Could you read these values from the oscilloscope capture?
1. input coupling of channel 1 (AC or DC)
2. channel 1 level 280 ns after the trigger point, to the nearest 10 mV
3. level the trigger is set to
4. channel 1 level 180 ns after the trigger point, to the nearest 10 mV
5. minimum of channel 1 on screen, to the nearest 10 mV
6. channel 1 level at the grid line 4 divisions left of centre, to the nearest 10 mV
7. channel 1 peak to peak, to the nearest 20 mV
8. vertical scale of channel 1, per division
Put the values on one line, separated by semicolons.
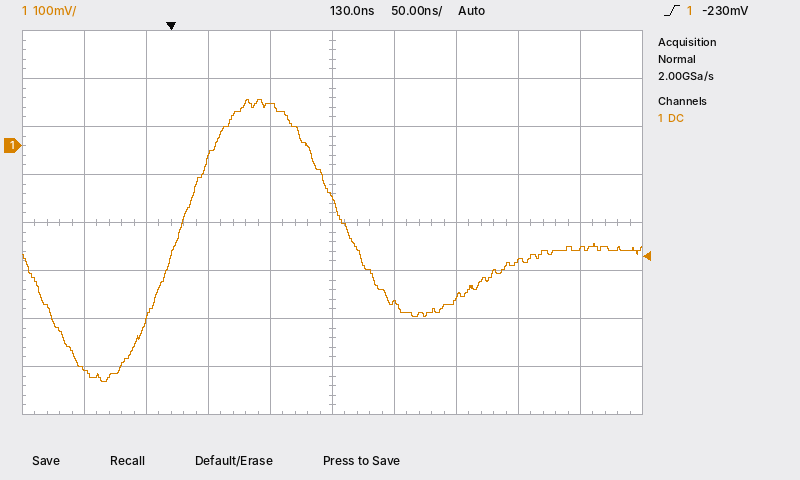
DC; -240 mV; -230 mV; -330 mV; -490 mV; -460 mV; 580 mV; 100 mV
